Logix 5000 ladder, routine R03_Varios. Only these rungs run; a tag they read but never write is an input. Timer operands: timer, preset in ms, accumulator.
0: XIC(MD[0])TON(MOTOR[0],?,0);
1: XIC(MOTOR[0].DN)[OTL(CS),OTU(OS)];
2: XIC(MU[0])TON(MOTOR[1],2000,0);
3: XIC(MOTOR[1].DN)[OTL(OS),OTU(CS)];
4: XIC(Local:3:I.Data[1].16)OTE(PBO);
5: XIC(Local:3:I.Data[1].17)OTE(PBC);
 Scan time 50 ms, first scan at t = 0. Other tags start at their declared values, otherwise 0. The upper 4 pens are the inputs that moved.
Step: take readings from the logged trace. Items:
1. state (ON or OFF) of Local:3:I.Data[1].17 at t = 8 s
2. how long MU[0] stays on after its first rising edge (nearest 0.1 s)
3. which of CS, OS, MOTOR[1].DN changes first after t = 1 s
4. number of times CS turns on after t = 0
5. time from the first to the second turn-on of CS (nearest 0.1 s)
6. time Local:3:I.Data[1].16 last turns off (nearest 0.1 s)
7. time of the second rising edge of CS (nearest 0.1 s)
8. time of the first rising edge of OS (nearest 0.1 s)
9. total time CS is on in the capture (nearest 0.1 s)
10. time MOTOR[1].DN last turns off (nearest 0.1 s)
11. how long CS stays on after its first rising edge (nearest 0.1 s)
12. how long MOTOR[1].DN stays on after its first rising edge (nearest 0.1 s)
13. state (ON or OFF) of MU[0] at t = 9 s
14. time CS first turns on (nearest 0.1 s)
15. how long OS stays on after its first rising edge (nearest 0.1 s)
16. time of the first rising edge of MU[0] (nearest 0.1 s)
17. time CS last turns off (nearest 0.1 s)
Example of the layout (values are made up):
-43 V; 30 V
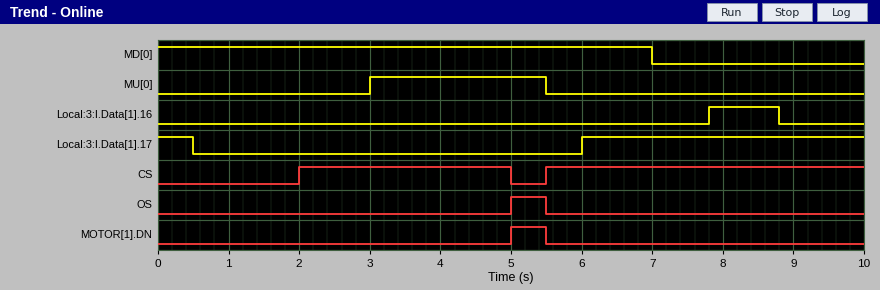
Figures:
ON; 2.5 s; CS; 2; 3.5 s; 8.8 s; 5.5 s; 5.0 s; 7.5 s; 5.5 s; 3.0 s; 0.5 s; OFF; 2.0 s; 0.5 s; 3.0 s; 5.0 s
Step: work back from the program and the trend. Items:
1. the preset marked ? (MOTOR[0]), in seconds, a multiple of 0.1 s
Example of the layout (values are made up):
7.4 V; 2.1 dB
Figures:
2.0 s
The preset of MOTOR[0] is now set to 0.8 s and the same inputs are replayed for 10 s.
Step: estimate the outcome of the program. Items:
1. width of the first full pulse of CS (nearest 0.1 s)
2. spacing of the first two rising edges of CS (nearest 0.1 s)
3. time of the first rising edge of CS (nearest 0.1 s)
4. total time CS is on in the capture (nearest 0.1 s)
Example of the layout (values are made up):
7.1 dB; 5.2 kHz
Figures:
4.2 s; 4.7 s; 0.8 s; 8.7 s
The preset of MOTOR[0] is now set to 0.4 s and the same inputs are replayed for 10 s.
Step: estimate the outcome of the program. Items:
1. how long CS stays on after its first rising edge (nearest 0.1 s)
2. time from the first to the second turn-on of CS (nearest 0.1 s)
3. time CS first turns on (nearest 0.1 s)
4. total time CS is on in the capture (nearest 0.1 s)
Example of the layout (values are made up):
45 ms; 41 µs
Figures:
4.6 s; 5.1 s; 0.4 s; 9.1 s
